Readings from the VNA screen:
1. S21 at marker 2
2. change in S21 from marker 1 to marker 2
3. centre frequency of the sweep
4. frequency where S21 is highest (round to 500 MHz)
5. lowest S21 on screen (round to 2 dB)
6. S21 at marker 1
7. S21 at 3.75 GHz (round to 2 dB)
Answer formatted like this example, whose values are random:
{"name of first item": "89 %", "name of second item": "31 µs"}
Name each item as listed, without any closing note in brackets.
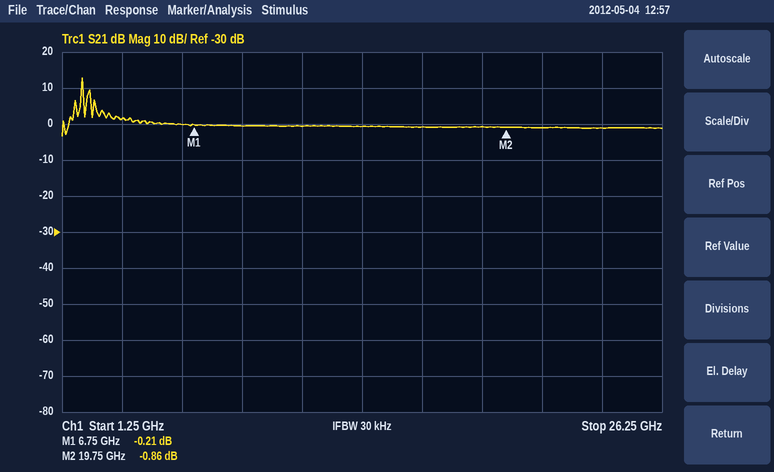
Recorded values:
{"S21 at marker 2": "-0.86 dB", "change in S21 from marker 1 to marker 2": "-0.65 dB", "centre frequency of the sweep": "13.75 GHz", "frequency where S21 is highest": "2.0 GHz", "lowest S21 on screen": "-4 dB", "S21 at marker 1": "-0.21 dB", "S21 at 3.75 GHz": "2 dB"}
